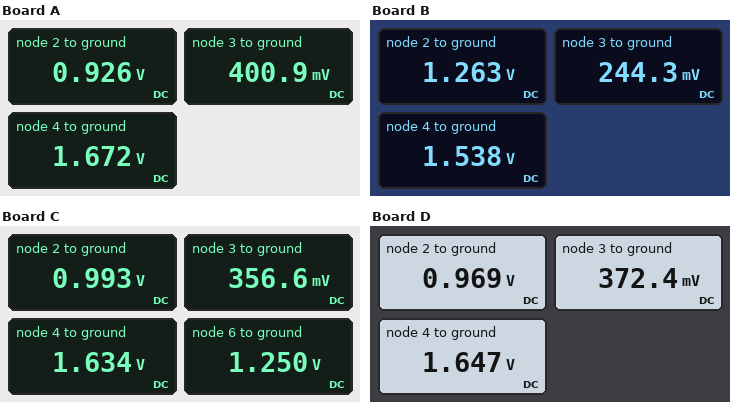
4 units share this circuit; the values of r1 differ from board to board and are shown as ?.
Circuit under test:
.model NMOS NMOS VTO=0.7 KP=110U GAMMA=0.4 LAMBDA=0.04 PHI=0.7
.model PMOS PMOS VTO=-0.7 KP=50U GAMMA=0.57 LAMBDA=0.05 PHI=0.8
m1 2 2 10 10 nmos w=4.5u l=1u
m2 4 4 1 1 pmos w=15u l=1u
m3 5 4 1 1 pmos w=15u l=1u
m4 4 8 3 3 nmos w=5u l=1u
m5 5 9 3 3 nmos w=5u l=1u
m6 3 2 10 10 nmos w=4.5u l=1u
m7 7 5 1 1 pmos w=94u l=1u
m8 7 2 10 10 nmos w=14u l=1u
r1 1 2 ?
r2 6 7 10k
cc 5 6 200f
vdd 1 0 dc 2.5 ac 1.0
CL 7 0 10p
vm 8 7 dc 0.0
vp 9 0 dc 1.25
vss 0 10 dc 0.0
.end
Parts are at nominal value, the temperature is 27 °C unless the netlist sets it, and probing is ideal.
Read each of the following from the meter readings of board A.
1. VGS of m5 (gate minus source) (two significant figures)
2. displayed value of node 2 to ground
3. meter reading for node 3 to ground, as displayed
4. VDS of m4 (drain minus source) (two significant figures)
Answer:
850 mV
0.926 V
400.9 mV
1.3 V
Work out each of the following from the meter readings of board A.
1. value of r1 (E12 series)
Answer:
120 kΩ
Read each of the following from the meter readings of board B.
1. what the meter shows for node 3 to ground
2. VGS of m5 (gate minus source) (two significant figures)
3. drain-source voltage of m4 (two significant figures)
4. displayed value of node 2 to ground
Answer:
244.3 mV
1.0 V
1.3 V
1.263 V
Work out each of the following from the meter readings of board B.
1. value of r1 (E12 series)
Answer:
15 kΩ
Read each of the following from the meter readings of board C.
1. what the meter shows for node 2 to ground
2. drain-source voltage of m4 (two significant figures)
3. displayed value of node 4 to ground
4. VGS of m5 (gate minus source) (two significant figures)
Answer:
0.993 V
1.3 V
1.634 V
890 mV
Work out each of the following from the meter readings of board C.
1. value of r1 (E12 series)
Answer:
68 kΩ
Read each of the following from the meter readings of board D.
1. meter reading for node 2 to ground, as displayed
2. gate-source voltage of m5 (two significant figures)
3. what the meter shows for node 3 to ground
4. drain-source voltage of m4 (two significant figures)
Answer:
0.969 V
880 mV
372.4 mV
1.3 V
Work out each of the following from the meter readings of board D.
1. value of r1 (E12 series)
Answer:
82 kΩ
